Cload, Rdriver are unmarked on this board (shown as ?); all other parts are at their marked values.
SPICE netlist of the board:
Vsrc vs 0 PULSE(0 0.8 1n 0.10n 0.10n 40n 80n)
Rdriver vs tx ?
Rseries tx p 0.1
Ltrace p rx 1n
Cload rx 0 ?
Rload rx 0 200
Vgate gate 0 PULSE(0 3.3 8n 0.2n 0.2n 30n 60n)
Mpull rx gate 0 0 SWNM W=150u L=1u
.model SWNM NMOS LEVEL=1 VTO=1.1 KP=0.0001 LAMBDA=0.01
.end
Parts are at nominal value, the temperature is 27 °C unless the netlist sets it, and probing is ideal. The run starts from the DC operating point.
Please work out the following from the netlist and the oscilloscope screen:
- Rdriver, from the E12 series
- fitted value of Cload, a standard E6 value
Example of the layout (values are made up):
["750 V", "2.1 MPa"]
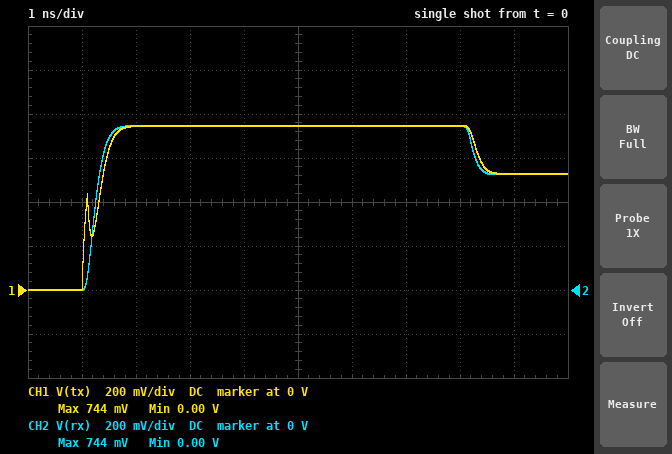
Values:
["15 Ω", "15 pF"]
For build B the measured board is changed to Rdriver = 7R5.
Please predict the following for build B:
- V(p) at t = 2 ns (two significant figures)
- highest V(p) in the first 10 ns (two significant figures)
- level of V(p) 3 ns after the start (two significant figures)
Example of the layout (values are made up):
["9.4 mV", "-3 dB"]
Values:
["760 mV", "840 mV", "770 mV"]
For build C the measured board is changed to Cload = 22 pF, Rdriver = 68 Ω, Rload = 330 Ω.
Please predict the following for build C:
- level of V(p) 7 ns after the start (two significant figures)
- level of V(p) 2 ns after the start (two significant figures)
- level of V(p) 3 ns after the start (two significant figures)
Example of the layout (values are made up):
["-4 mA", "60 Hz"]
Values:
["660 mV", "350 mV", "520 mV"]
